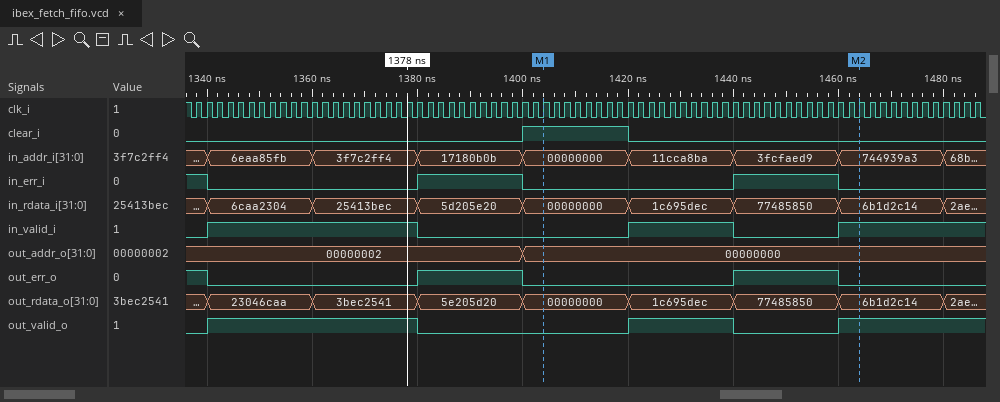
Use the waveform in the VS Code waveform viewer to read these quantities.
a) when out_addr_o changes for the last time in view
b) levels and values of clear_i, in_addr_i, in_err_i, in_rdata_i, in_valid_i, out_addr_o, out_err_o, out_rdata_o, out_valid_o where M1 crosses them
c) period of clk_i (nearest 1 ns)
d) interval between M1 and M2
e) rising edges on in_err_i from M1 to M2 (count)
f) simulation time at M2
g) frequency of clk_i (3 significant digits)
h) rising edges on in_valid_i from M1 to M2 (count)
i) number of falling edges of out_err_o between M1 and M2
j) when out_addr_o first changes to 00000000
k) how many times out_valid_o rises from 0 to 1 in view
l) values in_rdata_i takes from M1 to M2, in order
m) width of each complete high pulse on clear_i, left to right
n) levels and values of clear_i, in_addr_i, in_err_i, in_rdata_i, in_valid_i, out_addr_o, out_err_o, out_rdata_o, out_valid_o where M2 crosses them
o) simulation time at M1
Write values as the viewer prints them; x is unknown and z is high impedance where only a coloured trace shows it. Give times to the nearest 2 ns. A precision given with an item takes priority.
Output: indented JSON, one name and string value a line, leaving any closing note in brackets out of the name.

{
  "when out_addr_o changes for the last time in view": "1400 ns",
  "levels and values of clear_i, in_addr_i, in_err_i, in_rdata_i, in_valid_i, out_addr_o, out_err_o, out_rdata_o, out_valid_o where M1 crosses them": "clear_i=1, in_addr_i=00000000, in_err_i=0, in_rdata_i=00000000, in_valid_i=0, out_addr_o=00000000, out_err_o=0, out_rdata_o=00000000, out_valid_o=0",
  "period of clk_i": "2 ns",
  "interval between M1 and M2": "60 ns",
  "rising edges on in_err_i from M1 to M2": "1",
  "simulation time at M2": "1464 ns",
  "frequency of clk_i": "500 MHz",
  "rising edges on in_valid_i from M1 to M2": "2",
  "number of falling edges of out_err_o between M1 and M2": "1",
  "when out_addr_o first changes to 00000000": "1400 ns",
  "how many times out_valid_o rises from 0 to 1 in view": "3",
  "values in_rdata_i takes from M1 to M2, in order": "00000000, 1c695dec, 77485850, 6b1d2c14",
  "width of each complete high pulse on clear_i, left to right": "20 ns",
  "levels and values of clear_i, in_addr_i, in_err_i, in_rdata_i, in_valid_i, out_addr_o, out_err_o, out_rdata_o, out_valid_o where M2 crosses them": "clear_i=0, in_addr_i=744939a3, in_err_i=0, in_rdata_i=6b1d2c14, in_valid_i=1, out_addr_o=00000000, out_err_o=0, out_rdata_o=6b1d2c14, out_valid_o=1",
  "simulation time at M1": "1404 ns"
}
